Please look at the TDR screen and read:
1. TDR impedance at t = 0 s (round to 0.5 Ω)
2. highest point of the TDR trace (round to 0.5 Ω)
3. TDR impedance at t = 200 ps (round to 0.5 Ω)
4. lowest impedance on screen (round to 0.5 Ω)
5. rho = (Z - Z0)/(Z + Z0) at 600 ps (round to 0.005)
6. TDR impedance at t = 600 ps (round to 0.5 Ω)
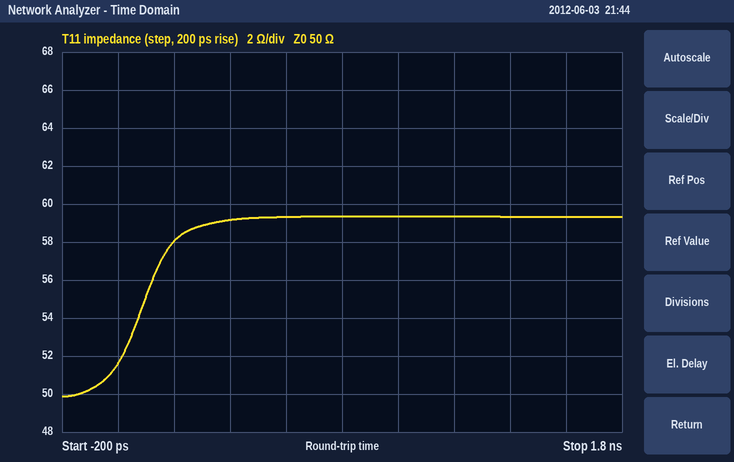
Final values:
51.5 Ω
59.5 Ω
58.0 Ω
50.0 Ω
+0.085
59.5 Ω
